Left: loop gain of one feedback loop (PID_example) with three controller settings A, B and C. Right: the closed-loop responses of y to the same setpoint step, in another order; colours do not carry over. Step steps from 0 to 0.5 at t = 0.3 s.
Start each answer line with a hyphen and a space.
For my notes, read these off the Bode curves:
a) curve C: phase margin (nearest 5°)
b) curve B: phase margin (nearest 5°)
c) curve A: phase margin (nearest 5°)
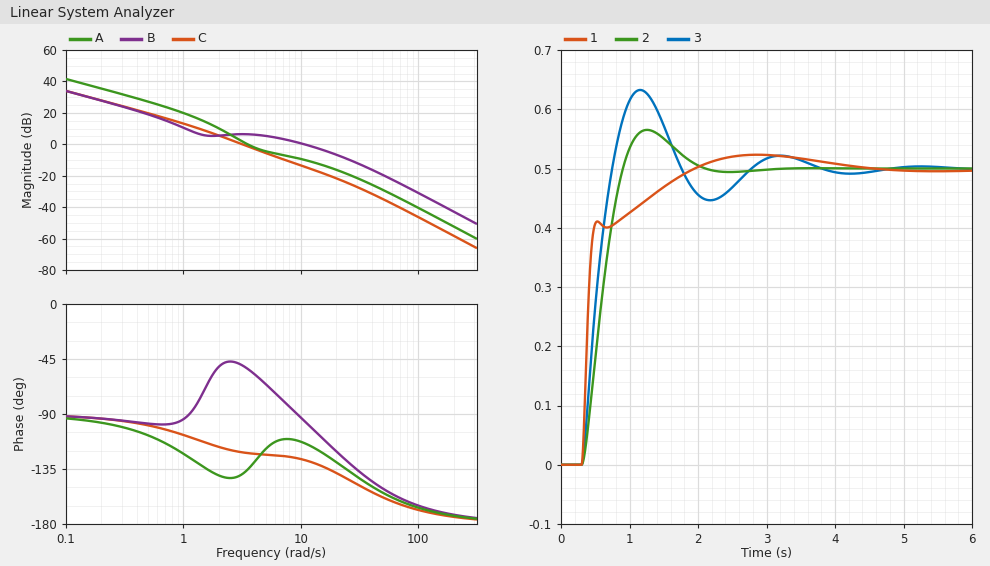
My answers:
- 60°
- 85°
- 45°
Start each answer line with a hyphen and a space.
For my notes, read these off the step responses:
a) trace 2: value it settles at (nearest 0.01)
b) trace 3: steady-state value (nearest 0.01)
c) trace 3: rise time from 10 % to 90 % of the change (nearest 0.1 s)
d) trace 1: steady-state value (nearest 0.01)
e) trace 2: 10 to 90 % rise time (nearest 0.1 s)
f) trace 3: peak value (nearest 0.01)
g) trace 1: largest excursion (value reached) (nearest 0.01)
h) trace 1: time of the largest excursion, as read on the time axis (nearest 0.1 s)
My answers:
- 0.50
- 0.50
- 0.3 s
- 0.50
- 0.4 s
- 0.63
- 0.52
- 2.9 s
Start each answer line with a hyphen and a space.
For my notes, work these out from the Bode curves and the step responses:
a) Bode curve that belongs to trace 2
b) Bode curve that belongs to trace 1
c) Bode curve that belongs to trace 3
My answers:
- C
- B
- A
